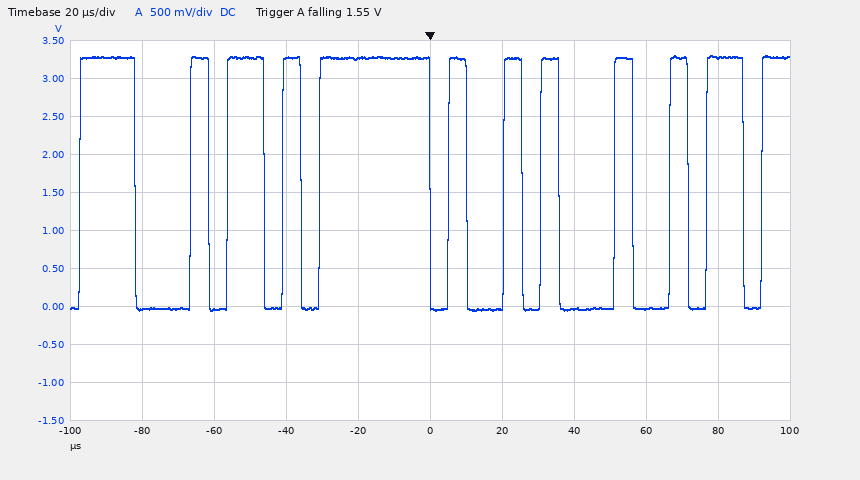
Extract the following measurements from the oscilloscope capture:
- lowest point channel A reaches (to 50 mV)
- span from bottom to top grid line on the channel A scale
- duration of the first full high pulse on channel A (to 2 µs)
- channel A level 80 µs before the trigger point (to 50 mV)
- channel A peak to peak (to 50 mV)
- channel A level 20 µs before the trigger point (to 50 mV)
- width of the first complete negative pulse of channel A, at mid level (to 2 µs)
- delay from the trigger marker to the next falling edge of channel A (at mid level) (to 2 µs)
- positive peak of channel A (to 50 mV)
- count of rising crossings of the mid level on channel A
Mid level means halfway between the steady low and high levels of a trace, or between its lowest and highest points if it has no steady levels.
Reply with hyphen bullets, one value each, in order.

- -50 mV
- 5 V
- 16 µs
- -50 mV
- 3.35 V
- 3.25 V
- 16 µs
- 10 µs
- 3.30 V
- 12
